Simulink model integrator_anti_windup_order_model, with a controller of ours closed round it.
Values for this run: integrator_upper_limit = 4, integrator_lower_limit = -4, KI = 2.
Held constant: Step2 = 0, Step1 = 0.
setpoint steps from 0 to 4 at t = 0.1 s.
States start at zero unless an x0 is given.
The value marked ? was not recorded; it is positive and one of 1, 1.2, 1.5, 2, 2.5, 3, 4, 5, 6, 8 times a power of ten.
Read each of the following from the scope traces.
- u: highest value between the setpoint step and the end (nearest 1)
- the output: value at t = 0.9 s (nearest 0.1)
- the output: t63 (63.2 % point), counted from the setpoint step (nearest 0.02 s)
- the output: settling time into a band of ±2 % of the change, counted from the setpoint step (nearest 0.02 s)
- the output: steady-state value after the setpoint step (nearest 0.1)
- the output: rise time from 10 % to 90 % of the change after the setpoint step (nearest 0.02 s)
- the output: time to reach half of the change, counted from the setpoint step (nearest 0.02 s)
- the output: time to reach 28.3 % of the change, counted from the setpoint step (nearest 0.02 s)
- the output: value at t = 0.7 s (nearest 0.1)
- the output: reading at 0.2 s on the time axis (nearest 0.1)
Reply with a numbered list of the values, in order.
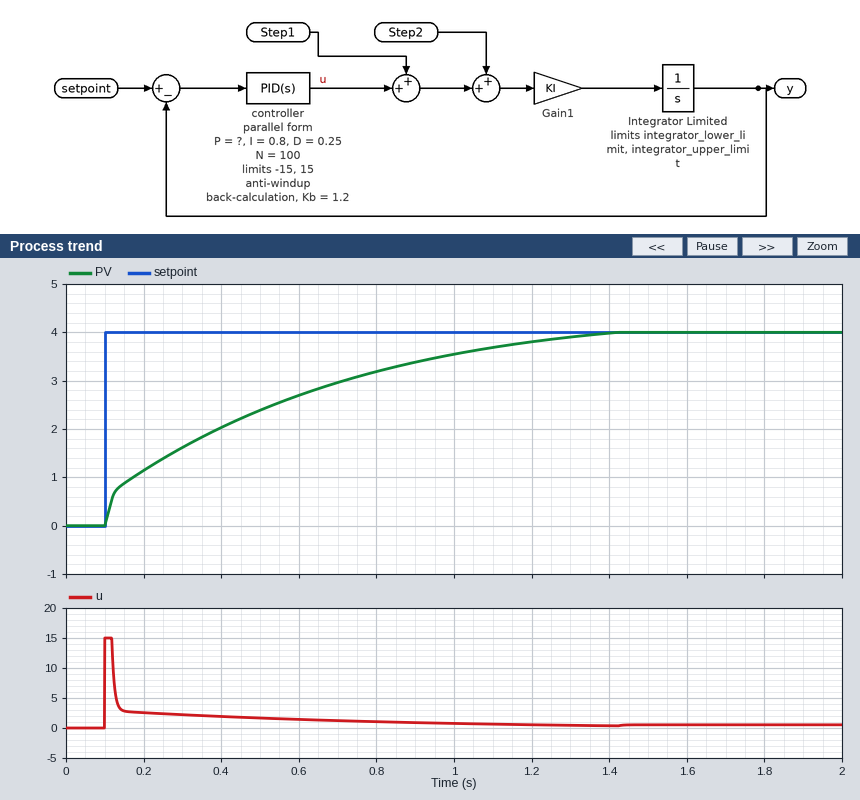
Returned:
1. 15
2. 3.4
3. 0.44 s
4. 1.22 s
5. 4.0
6. 0.92 s
7. 0.30 s
8. 0.10 s
9. 3.0
10. 1.1
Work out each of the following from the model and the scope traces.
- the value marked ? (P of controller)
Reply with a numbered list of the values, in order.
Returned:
1. 1.5
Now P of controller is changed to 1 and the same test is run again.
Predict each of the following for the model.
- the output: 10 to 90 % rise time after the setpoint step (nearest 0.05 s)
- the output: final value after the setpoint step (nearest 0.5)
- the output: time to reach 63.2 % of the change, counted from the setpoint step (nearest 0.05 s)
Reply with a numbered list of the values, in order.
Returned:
1. 1.10 s
2. 4.0
3. 0.60 s
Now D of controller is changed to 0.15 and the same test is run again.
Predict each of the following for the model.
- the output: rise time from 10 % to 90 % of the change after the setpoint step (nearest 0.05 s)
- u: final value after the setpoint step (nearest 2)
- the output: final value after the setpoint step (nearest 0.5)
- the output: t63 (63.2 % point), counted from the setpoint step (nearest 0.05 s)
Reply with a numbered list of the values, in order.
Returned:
1. 0.75 s
2. 0
3. 4.0
4. 0.35 s
